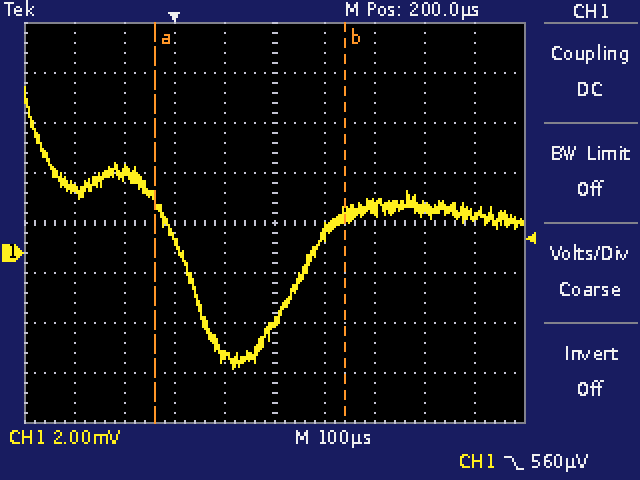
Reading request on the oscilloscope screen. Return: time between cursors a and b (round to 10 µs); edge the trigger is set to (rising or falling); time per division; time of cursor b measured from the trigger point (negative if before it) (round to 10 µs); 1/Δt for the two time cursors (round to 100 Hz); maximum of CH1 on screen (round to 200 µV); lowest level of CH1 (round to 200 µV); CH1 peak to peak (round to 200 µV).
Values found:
380 µs
falling
100 µs
+340 µs
2.6 kHz
6.6 mV
-4.6 mV
11.2 mV
